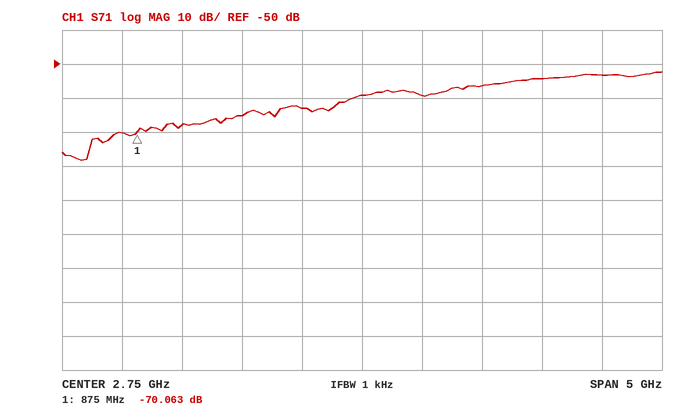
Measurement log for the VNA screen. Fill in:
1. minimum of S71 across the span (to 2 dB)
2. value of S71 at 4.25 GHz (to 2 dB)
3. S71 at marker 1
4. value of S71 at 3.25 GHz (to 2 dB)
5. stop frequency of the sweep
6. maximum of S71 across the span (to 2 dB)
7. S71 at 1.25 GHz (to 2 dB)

-78 dB
-54 dB
-70.063 dB
-60 dB
5.25 GHz
-52 dB
-68 dB
